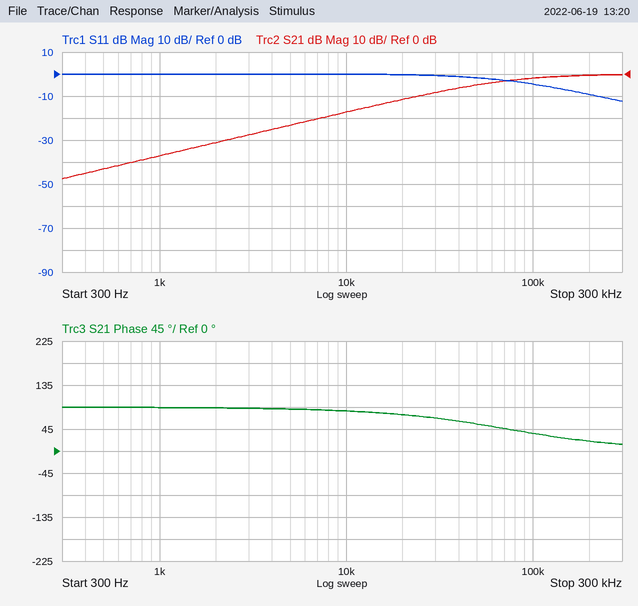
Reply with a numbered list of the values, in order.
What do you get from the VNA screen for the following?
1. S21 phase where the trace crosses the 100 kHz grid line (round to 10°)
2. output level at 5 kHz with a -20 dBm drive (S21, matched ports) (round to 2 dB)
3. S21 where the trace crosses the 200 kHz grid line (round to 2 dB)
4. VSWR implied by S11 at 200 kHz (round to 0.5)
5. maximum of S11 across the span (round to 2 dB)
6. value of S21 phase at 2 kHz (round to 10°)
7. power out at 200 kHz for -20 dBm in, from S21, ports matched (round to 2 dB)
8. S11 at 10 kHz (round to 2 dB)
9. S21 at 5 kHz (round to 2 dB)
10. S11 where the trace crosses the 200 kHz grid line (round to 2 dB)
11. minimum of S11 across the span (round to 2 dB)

1. 40°
2. -44 dBm
3. 0 dB
4. 2.0
5. 0 dB
6. 90°
7. -20 dBm
8. 0 dB
9. -24 dB
10. -10 dB
11. -12 dB
